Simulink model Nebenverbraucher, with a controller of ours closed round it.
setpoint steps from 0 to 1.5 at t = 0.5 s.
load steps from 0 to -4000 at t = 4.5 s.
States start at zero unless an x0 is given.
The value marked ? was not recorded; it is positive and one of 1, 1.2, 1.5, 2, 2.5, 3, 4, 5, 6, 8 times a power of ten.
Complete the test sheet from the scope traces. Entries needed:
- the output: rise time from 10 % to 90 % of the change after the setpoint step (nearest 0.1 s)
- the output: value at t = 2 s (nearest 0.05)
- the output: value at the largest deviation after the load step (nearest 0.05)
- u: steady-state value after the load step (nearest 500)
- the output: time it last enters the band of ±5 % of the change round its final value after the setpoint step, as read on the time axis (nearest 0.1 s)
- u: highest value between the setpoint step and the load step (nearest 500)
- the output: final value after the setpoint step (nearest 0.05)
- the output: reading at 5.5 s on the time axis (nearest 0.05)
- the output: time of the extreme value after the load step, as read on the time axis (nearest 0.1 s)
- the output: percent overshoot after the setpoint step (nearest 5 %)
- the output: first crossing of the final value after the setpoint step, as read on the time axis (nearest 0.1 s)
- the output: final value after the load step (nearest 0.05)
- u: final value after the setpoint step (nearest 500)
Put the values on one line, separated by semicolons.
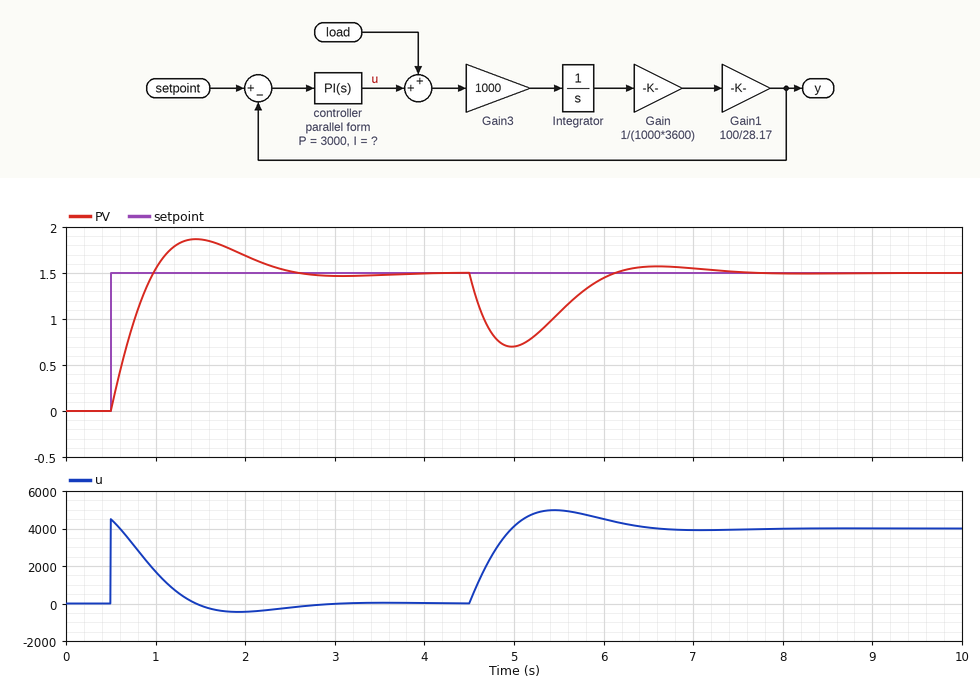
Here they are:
0.4 s; 1.70; 0.70; 4000; 2.3 s; 4500; 1.50; 1.05; 5.0 s; 25 %; 1.0 s; 1.50; 0
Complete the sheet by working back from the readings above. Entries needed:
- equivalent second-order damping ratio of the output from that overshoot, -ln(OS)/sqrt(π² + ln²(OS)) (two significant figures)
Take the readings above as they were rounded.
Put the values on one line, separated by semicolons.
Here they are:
0.40
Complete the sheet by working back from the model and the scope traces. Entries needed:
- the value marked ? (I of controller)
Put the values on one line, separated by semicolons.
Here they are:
6000
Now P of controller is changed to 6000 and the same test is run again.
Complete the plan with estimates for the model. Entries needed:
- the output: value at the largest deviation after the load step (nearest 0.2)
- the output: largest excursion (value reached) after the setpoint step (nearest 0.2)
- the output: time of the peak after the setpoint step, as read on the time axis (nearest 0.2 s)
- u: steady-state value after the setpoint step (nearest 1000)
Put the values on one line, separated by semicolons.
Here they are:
1.0; 1.6; 1.2 s; 0
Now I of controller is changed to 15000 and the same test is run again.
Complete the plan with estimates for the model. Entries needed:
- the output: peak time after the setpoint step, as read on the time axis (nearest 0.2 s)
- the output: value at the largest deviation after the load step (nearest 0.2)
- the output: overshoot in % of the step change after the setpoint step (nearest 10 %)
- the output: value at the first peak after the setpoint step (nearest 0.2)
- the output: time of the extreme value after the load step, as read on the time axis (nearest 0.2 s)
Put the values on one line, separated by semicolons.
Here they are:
1.2 s; 0.8; 40 %; 2.0; 4.8 s
